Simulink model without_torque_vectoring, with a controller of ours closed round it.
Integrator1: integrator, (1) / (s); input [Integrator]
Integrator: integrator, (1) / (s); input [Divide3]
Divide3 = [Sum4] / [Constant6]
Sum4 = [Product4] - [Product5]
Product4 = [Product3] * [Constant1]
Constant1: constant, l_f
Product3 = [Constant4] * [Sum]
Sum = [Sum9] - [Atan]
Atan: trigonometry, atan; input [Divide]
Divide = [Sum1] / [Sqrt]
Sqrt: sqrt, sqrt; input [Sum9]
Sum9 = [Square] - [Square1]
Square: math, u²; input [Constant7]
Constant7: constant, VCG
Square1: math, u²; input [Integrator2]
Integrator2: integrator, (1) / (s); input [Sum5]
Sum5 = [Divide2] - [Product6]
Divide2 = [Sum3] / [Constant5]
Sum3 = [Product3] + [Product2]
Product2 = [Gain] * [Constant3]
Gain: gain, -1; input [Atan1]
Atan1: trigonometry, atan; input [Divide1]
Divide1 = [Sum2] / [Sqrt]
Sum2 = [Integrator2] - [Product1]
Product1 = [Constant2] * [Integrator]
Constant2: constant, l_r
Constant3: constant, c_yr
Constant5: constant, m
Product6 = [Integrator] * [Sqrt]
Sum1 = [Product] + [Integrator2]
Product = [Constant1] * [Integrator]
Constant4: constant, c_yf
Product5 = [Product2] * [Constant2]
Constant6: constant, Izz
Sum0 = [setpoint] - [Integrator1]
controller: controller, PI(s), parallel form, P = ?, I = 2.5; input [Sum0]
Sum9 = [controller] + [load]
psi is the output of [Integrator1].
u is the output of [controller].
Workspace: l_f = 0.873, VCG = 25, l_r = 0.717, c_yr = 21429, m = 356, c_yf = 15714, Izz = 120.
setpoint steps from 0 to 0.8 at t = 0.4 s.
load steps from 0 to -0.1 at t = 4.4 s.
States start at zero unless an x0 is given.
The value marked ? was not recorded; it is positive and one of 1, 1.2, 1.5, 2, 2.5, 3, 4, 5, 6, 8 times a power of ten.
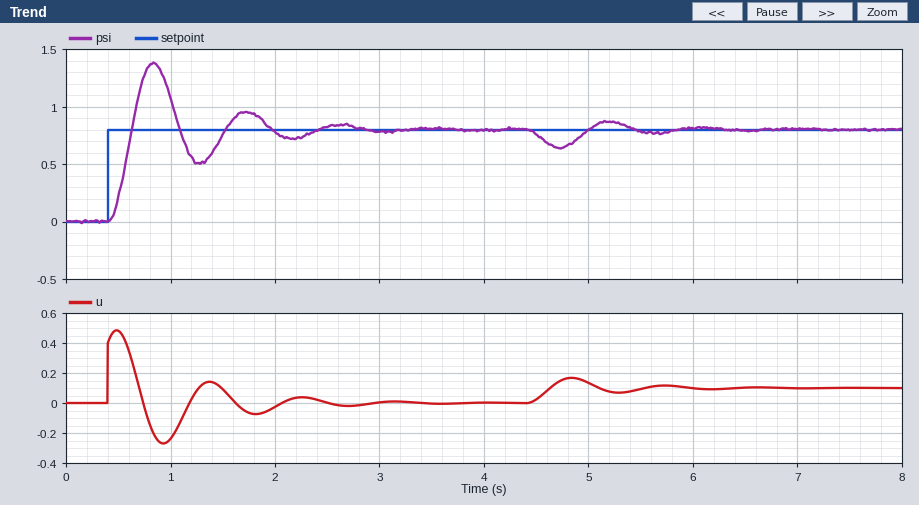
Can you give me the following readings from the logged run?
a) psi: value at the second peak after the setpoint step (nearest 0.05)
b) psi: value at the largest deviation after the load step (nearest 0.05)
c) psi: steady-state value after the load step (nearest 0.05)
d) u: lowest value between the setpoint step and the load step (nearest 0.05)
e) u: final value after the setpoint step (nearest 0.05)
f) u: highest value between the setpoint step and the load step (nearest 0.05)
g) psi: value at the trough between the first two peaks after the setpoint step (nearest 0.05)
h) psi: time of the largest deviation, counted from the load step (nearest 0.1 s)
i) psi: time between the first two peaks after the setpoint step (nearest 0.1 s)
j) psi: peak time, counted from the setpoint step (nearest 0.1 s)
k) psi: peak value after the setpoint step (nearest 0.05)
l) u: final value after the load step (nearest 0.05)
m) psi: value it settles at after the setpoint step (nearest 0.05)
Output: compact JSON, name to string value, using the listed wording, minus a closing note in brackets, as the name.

{"psi: value at the second peak after the setpoint step": "0.95", "psi: value at the largest deviation after the load step": "0.65", "psi: steady-state value after the load step": "0.80", "u: lowest value between the setpoint step and the load step": "-0.25", "u: final value after the setpoint step": "0.00", "u: highest value between the setpoint step and the load step": "0.50", "psi: value at the trough between the first two peaks after the setpoint step": "0.50", "psi: time of the largest deviation, counted from the load step": "0.3 s", "psi: time between the first two peaks after the setpoint step": "0.9 s", "psi: peak time, counted from the setpoint step": "0.4 s", "psi: peak value after the setpoint step": "1.40", "u: final value after the load step": "0.10", "psi: value it settles at after the setpoint step": "0.80"}
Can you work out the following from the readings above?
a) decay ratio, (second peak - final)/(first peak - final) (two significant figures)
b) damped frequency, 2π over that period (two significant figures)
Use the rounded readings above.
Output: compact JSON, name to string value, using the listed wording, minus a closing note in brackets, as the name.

{"decay ratio, (second peak - final)/(first peak - final)": "0.25", "damped frequency, 2π over that period": "7.0 rad/s"}
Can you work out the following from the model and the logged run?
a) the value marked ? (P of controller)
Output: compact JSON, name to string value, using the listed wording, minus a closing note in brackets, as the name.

{"the value marked ?": "0.5"}
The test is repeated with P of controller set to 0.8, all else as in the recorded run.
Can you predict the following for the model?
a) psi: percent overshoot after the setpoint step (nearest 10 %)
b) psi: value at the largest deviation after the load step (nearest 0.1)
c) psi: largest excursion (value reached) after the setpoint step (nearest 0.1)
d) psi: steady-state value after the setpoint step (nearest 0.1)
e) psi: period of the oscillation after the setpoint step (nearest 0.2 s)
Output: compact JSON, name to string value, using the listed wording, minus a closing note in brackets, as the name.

{"psi: percent overshoot after the setpoint step": "60 %", "psi: value at the largest deviation after the load step": "0.7", "psi: largest excursion (value reached) after the setpoint step": "1.3", "psi: steady-state value after the setpoint step": "0.8", "psi: period of the oscillation after the setpoint step": "0.6 s"}
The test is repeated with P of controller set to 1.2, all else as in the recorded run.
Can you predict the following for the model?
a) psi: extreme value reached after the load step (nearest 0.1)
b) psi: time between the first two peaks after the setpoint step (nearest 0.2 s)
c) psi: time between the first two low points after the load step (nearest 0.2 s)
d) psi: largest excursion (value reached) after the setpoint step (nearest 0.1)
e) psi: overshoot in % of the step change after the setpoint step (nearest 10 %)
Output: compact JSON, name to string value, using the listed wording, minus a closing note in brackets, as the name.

{"psi: extreme value reached after the load step": "0.7", "psi: time between the first two peaks after the setpoint step": "0.6 s", "psi: time between the first two low points after the load step": "0.6 s", "psi: largest excursion (value reached) after the setpoint step": "1.2", "psi: overshoot in % of the step change after the setpoint step": "50 %"}
